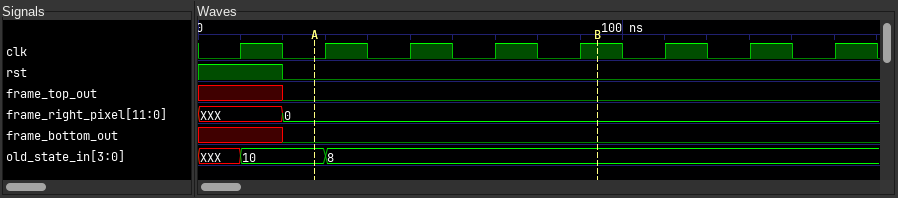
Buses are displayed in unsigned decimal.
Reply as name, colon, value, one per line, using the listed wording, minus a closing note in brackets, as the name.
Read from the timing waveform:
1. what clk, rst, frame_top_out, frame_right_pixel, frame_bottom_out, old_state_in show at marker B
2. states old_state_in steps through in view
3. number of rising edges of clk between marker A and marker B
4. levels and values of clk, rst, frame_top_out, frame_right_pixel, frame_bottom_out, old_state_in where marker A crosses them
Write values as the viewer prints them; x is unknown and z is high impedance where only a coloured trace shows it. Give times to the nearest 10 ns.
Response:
what clk, rst, frame_top_out, frame_right_pixel, frame_bottom_out, old_state_in show at marker B: clk=1, rst=0, frame_top_out=0, frame_right_pixel=0, frame_bottom_out=0, old_state_in=8
states old_state_in steps through in view: XXX, 10, 8
number of rising edges of clk between marker A and marker B: 4
levels and values of clk, rst, frame_top_out, frame_right_pixel, frame_bottom_out, old_state_in where marker A crosses them: clk=0, rst=0, frame_top_out=0, frame_right_pixel=0, frame_bottom_out=0, old_state_in=10
